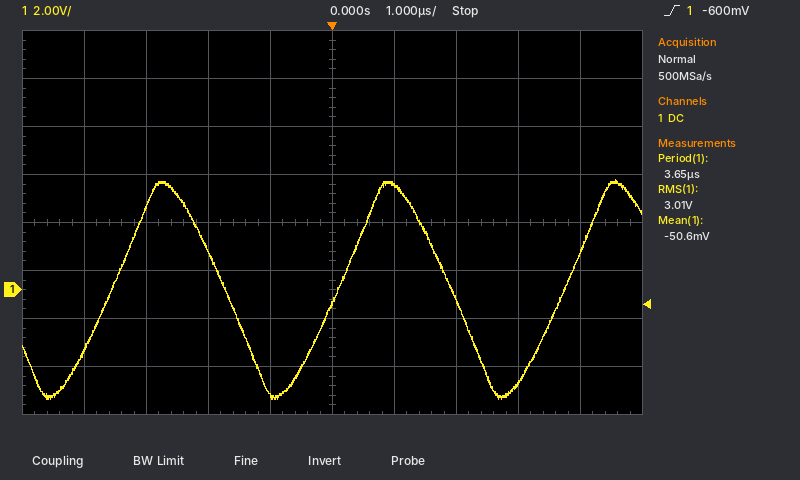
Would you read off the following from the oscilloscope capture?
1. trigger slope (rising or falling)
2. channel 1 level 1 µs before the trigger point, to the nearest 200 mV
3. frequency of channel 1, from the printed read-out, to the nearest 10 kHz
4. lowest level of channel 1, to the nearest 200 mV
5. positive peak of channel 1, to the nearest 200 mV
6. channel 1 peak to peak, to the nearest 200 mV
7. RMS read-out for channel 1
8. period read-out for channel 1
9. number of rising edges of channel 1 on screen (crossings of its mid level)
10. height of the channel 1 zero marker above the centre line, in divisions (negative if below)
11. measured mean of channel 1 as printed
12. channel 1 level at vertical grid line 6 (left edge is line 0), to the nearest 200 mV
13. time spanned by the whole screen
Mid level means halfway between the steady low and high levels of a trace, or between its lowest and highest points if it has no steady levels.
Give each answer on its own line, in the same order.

rising
-4.4 V
270 kHz
-4.6 V
4.6 V
9.2 V
3.01 V
3.65 µs
3
-1.4 div
-50.6 mV
4.4 V
10 µs
